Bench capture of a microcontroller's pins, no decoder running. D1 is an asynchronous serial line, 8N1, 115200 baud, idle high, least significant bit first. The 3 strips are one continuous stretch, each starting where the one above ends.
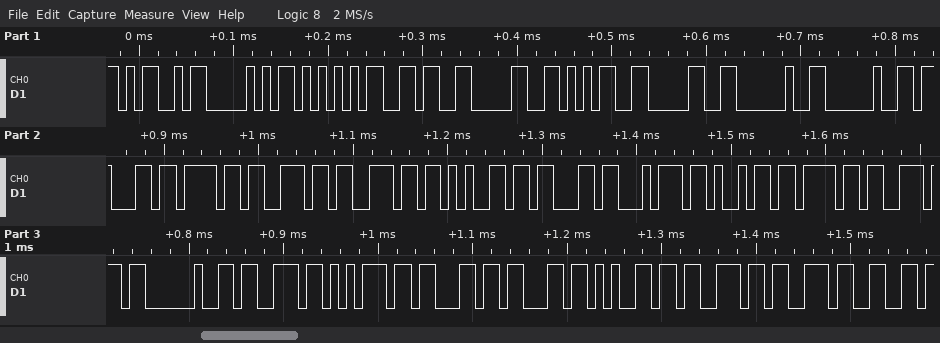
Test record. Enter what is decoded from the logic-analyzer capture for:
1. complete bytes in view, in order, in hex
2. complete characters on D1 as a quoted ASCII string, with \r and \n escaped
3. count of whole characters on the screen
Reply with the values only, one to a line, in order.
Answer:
4D 50 55 36 30 35 30 20 20 63 6F 6E 6E 65 63 74 69 6F 6E 20 73 75 63 63 65 73 73 66
"MPU6050  connection successf"
28
